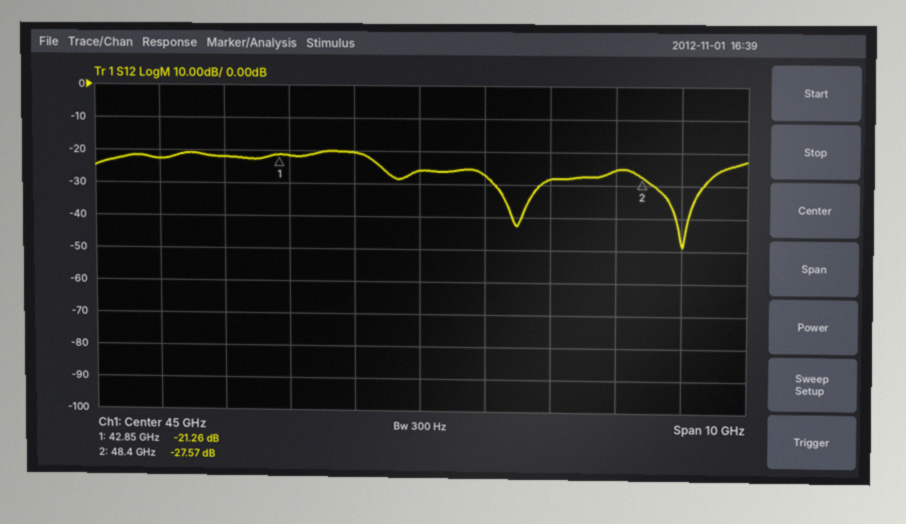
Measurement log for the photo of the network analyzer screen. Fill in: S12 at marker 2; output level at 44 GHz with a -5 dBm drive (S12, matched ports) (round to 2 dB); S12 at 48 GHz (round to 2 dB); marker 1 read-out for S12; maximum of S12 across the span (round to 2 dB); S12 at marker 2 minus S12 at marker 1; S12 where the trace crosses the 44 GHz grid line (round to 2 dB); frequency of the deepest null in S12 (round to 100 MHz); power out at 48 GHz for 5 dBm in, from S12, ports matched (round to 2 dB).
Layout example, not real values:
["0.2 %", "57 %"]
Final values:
["-27.57 dB", "-26 dBm", "-26 dB", "-21.26 dB", "-20 dB", "-6.31 dB", "-20 dB", "49.0 GHz", "-20 dBm"]
